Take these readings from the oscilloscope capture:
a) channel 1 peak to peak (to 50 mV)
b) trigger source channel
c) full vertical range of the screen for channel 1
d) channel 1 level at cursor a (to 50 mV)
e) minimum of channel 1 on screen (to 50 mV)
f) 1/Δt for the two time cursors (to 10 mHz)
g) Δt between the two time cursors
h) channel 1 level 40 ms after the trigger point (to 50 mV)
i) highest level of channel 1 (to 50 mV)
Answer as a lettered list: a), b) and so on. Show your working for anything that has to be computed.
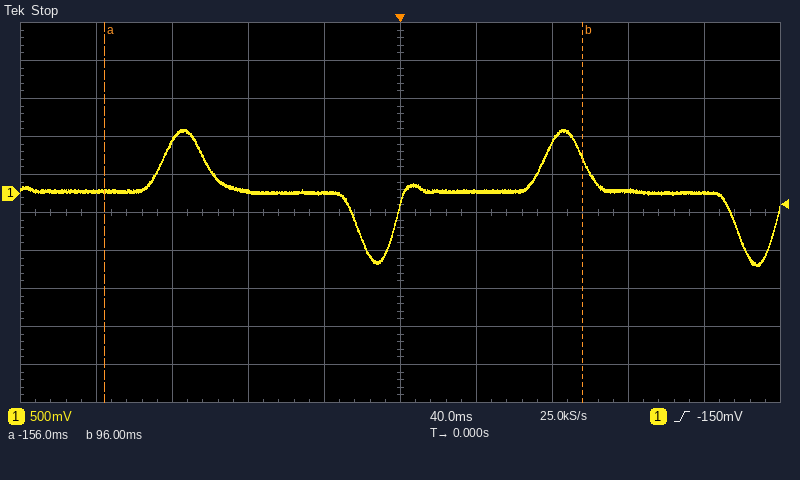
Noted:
a) 850 mV − (-950 mV) = 1.80 V
b) channel 1
c) 5 V
d) 50 mV
e) -950 mV
f) 1 / 252 ms ≈ 3.97 Hz
g) 96 ms − (-156 ms) = 252 ms
h) 50 mV
i) 850 mV
